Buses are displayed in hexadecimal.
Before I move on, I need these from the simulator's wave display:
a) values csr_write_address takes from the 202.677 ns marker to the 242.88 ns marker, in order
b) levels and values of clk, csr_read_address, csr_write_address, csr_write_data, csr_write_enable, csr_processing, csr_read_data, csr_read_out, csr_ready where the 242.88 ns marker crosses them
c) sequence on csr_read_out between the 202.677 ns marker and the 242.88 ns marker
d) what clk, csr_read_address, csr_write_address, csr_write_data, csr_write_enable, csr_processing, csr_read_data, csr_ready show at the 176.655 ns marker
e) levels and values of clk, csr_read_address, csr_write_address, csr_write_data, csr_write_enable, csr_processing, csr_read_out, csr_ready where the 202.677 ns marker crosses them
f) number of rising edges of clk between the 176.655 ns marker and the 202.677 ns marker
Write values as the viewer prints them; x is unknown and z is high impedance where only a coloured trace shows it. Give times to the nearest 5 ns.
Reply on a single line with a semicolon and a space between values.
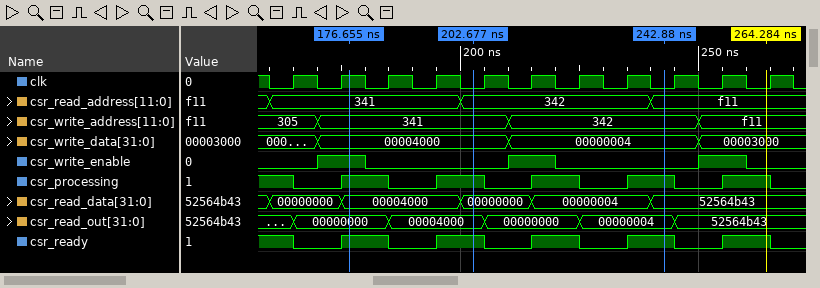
341, 342; clk=0, csr_read_address=f11, csr_write_address=342, csr_write_data=00000004, csr_write_enable=0, csr_processing=1, csr_read_data=52564b43, csr_read_out=00000004, csr_ready=1; 00004000, 00000000, 00000004; clk=1, csr_read_address=341, csr_write_address=341, csr_write_data=00004000, csr_write_enable=1, csr_processing=1, csr_read_data=00004000, csr_ready=1; clk=0, csr_read_address=342, csr_write_address=341, csr_write_data=00004000, csr_write_enable=0, csr_processing=1, csr_read_out=00004000, csr_ready=1; 2
